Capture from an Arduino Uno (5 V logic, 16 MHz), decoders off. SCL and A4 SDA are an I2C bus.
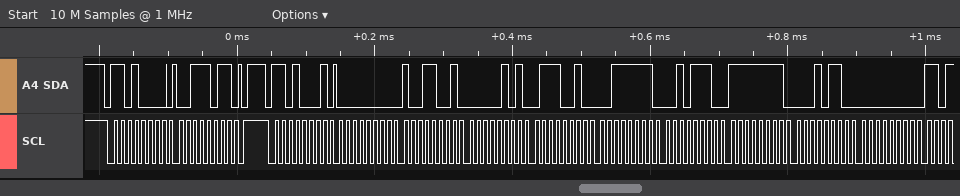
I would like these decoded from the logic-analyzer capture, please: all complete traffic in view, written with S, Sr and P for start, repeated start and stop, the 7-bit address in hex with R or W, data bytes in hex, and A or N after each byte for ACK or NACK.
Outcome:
S 68W A 3B A P S 68R A 00 A 99 A 05 A 72 A 3F A 2E A FF A 16 A 00 A
